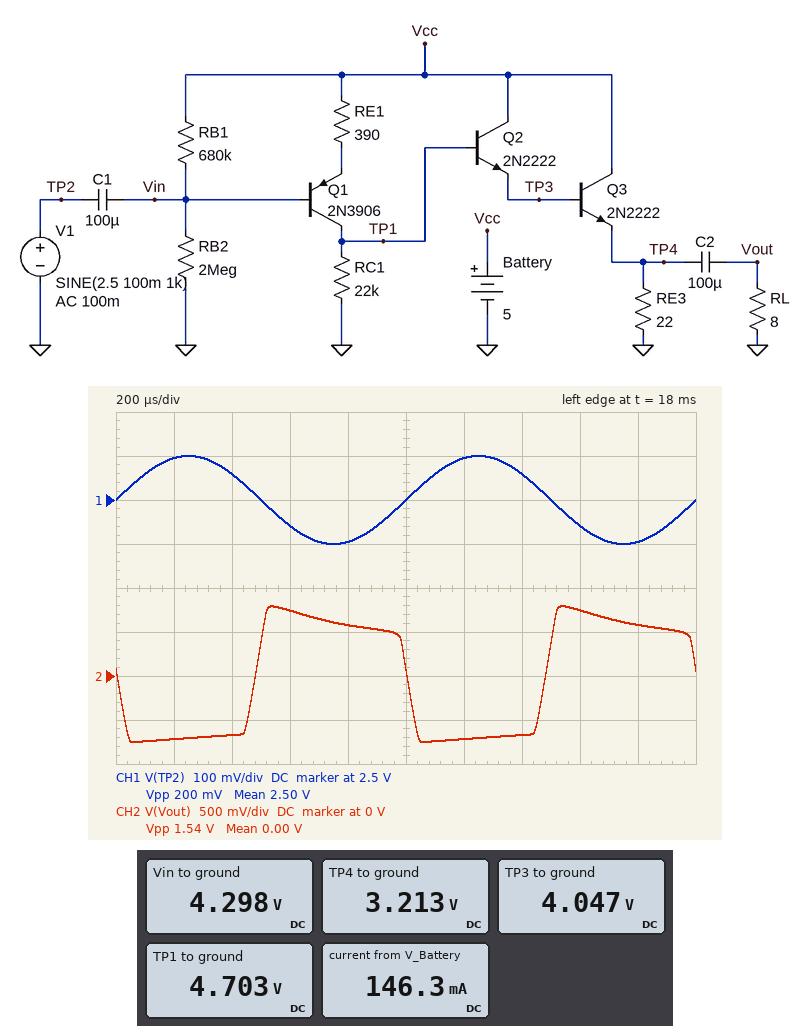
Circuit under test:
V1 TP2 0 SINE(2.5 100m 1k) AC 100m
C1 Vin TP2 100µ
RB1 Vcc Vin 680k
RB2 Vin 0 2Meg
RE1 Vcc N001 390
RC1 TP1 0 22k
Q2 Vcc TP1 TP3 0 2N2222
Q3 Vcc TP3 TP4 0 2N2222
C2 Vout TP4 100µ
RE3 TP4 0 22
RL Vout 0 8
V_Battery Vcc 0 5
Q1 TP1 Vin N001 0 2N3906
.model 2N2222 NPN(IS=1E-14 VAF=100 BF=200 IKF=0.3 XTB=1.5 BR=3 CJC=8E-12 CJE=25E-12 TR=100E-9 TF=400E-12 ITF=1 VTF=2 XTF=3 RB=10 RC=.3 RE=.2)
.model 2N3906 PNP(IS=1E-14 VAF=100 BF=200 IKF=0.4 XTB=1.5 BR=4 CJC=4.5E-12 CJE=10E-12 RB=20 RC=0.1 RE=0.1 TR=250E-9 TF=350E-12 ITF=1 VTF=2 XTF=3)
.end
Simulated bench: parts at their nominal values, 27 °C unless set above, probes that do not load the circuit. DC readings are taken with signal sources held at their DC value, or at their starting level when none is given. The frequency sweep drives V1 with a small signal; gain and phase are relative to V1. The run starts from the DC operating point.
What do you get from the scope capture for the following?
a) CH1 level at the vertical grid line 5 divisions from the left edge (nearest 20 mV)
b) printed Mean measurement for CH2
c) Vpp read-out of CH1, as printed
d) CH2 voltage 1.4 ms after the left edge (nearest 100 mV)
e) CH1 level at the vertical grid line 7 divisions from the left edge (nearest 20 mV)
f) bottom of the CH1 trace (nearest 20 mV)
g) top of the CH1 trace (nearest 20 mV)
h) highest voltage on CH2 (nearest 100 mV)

2.50 V
0.00 V
200 mV
-700 mV
2.56 V
2.40 V
2.60 V
800 mV
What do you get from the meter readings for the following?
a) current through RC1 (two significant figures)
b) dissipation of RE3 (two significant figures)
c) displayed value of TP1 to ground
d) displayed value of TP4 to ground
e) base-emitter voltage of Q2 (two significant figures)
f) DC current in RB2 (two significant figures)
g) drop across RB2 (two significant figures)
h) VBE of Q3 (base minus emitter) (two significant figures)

210 µA
470 mW
4.703 V
3.213 V
660 mV
2.1 µA
4.3 V
830 mV
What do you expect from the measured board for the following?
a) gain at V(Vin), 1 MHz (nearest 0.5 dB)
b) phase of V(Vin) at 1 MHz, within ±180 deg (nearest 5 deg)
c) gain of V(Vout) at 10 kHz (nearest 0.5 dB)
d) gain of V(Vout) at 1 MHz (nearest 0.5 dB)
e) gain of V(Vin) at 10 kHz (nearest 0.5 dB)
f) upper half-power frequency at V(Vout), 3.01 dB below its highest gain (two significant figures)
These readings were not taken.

0 dB
0 deg
30.0 dB
23.5 dB
0 dB
550 kHz
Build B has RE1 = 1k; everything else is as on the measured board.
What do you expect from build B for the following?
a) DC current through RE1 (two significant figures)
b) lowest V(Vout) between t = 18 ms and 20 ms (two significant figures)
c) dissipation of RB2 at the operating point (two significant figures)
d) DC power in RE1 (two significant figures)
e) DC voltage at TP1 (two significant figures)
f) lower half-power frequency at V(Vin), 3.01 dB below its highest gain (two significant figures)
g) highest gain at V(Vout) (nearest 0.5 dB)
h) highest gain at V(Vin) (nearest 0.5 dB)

190 µA
-700 mV
8.8 µW
35 µW
4.0 V
10 mHz
23.5 dB
0 dB
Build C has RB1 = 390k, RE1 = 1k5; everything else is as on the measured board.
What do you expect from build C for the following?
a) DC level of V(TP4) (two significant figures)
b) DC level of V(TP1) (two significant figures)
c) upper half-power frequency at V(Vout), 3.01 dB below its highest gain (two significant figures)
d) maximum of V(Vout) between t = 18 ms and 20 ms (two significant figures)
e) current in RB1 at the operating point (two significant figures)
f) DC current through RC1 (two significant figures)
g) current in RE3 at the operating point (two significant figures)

310 mV
1.6 V
560 kHz
530 mV
1.8 µA
74 µA
14 mA
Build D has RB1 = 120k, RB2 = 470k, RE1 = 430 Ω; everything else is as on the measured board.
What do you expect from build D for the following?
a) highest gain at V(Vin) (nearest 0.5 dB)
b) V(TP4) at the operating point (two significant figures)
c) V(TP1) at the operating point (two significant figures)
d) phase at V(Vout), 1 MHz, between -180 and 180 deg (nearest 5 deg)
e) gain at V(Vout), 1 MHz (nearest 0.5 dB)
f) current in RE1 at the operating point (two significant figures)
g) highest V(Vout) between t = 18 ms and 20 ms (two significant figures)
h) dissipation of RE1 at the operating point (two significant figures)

0 dB
3.3 V
4.8 V
90 deg
8.0 dB
230 µA
750 mV
22 µW
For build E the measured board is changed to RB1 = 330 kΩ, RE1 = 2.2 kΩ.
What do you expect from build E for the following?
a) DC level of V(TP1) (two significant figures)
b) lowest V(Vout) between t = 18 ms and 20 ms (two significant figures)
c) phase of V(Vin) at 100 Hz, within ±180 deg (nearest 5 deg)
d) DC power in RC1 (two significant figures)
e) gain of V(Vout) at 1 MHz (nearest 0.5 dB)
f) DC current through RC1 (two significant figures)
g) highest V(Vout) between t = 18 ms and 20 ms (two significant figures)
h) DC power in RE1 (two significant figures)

850 mV
-39 mV
0 deg
33 µW
-57.5 dB
39 µA
150 mV
3.3 µW
